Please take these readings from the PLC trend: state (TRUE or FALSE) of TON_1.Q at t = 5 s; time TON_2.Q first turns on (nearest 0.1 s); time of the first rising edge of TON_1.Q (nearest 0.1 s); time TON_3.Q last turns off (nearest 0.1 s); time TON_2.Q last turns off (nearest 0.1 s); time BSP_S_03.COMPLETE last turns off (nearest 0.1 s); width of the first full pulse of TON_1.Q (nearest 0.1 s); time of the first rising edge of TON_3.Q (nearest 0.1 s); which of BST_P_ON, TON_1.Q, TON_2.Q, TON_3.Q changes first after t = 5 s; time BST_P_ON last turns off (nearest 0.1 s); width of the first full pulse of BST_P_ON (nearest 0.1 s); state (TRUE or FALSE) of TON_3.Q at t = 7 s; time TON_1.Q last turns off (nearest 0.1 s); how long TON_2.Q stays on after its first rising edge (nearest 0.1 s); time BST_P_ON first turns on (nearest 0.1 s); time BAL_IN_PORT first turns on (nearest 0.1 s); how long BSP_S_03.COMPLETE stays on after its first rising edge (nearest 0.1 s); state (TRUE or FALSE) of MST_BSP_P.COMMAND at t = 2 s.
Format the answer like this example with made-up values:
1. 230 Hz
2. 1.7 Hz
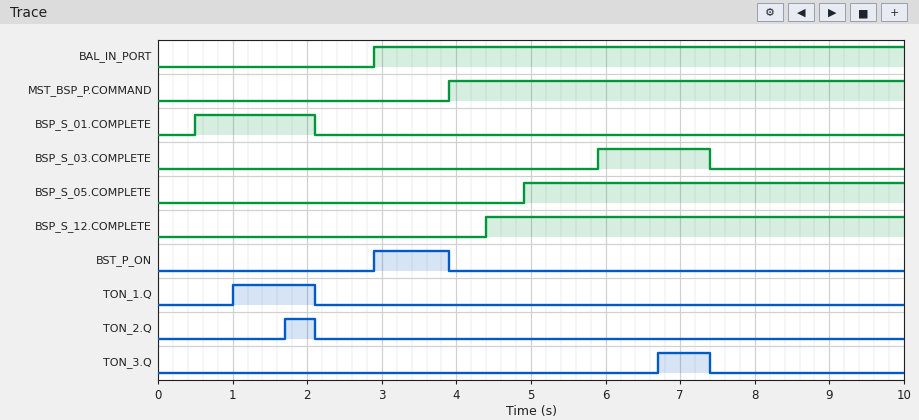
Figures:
1. FALSE
2. 1.7 s
3. 1.0 s
4. 7.4 s
5. 2.1 s
6. 7.4 s
7. 1.1 s
8. 6.7 s
9. TON_3.Q
10. 3.9 s
11. 1.0 s
12. TRUE
13. 2.1 s
14. 0.4 s
15. 2.9 s
16. 2.9 s
17. 1.5 s
18. FALSE
